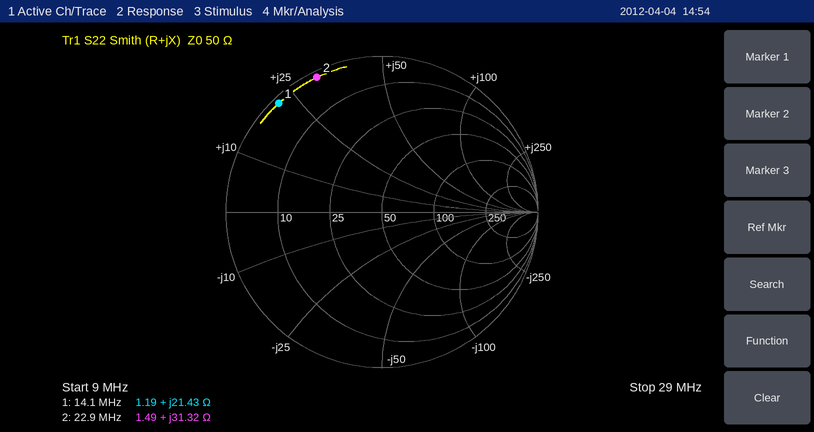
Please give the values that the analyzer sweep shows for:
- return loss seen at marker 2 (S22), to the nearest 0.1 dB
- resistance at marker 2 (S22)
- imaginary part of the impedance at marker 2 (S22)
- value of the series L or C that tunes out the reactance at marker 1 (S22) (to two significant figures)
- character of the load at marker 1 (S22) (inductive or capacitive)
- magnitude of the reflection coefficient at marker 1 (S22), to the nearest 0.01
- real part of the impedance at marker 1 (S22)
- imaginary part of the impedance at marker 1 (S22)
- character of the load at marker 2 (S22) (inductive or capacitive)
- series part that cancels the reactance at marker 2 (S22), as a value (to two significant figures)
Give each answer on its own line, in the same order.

0.4 dB
1.49 Ω
+31.32 Ω
530 pF
inductive
0.96
1.19 Ω
+21.43 Ω
inductive
220 pF
